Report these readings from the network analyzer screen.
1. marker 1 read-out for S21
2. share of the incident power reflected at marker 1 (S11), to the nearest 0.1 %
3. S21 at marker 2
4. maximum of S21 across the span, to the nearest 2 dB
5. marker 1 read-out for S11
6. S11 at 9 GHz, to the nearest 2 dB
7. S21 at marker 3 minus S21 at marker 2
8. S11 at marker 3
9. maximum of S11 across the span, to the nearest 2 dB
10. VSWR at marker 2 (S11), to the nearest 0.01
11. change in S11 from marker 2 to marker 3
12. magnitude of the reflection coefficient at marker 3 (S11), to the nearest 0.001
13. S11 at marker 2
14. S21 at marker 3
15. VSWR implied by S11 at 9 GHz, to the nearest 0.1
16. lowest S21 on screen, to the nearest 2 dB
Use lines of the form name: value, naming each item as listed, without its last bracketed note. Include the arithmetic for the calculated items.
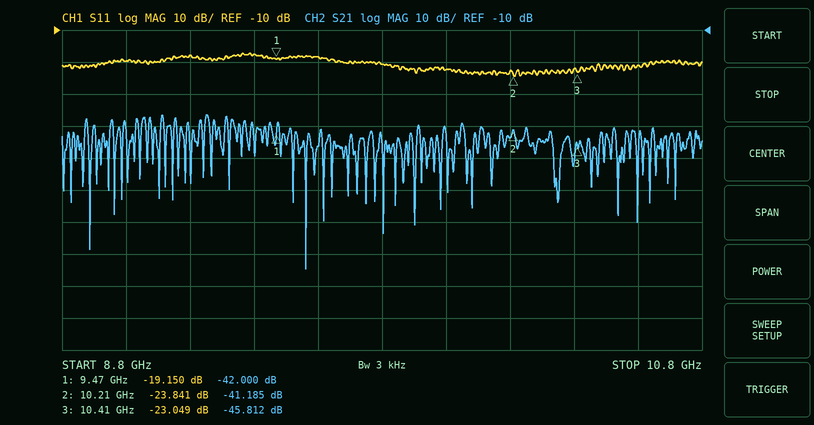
marker 1 read-out for S21: -42.000 dB
share of the incident power reflected at marker 1 (S11), to the nearest 0.1 %: 10^(-19.15/10) ≈ 1.2 %
S21 at marker 2: -41.185 dB
maximum of S21 across the span, to the nearest 2 dB: -36 dB
marker 1 read-out for S11: -19.150 dB
S11 at 9 GHz, to the nearest 2 dB: -20 dB
S21 at marker 3 minus S21 at marker 2: -45.812 − (-41.185) = -4.627 dB
S11 at marker 3: -23.049 dB
maximum of S11 across the span, to the nearest 2 dB: -18 dB
VSWR at marker 2 (S11), to the nearest 0.01: (1 + 0.0643)/(1 − 0.0643) ≈ 1.14
change in S11 from marker 2 to marker 3: -23.049 − (-23.841) = 0.792 dB
magnitude of the reflection coefficient at marker 3 (S11), to the nearest 0.001: 10^(-23.049/20) ≈ 0.070
S11 at marker 2: -23.841 dB
S21 at marker 3: -45.812 dB
VSWR implied by S11 at 9 GHz, to the nearest 0.1: |Γ| = 10^(-20/20) = 0.1000; VSWR = (1 + 0.1000)/(1 − 0.1000) ≈ 1.2
lowest S21 on screen, to the nearest 2 dB: -84 dB
